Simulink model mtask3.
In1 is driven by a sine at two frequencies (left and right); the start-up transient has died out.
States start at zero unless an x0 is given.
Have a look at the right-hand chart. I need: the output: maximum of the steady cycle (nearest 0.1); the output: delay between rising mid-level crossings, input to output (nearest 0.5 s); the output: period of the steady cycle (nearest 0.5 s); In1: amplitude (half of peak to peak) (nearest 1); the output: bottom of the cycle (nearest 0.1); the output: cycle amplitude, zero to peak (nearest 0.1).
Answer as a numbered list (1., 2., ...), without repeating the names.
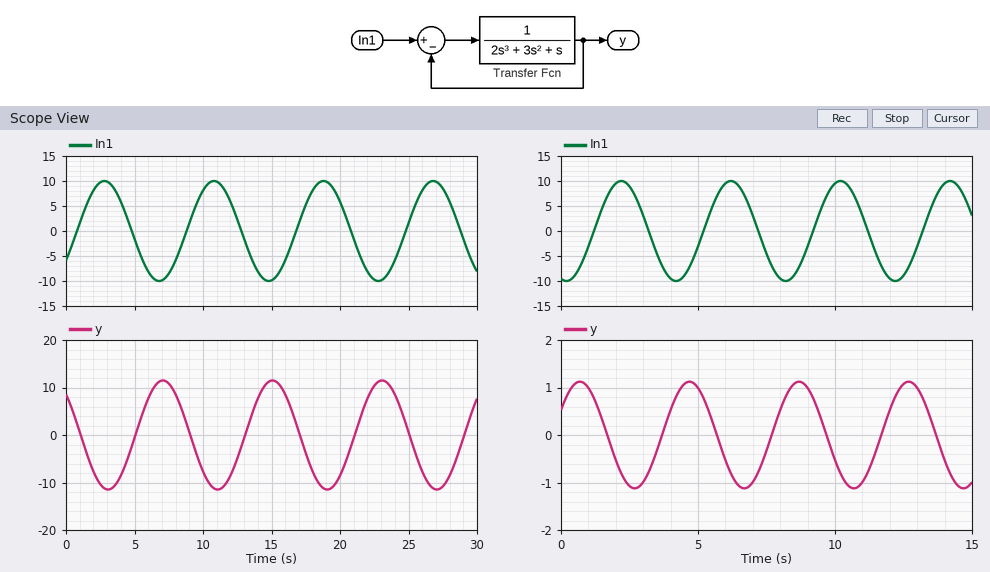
1. 1.1
2. 2.5 s
3. 4.0 s
4. 10
5. -1.1
6. 1.1
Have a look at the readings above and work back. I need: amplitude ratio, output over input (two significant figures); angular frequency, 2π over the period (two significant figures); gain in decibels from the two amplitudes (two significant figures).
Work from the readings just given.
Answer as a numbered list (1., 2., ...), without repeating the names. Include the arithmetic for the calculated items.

1. 1.1 / 10 = 0.11
2. 2π / 4 = 1.6 rad/s
3. 20 log10(1.1 / 10) = -19 dB
